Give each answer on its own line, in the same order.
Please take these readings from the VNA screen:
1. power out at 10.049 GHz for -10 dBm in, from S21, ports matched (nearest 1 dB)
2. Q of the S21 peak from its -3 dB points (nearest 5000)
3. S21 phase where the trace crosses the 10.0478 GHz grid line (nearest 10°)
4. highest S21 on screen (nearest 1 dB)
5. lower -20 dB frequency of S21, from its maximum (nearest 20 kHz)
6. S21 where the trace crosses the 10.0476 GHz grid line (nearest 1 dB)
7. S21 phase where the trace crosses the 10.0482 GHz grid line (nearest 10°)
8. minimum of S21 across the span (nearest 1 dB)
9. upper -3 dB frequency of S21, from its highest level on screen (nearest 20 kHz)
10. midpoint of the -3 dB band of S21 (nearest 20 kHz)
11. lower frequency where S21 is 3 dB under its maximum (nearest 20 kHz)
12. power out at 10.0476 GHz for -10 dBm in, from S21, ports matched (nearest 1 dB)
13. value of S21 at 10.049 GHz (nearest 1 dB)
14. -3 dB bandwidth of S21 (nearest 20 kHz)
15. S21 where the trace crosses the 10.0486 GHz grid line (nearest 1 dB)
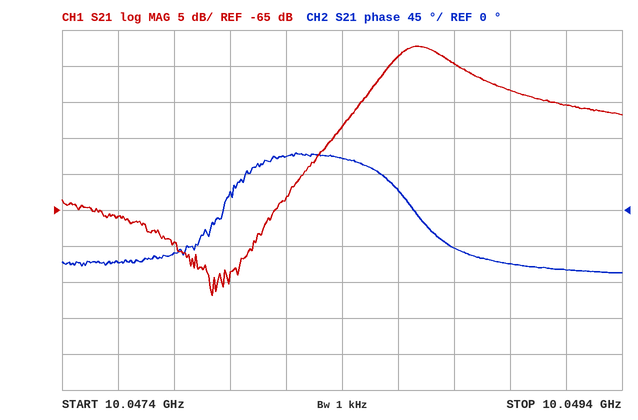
-58 dBm
40000
-50°
-42 dB
10.04822 GHz
-66 dB
70°
-77 dB
10.04882 GHz
10.04870 GHz
10.04856 GHz
-76 dBm
-48 dB
260 kHz
-44 dB
